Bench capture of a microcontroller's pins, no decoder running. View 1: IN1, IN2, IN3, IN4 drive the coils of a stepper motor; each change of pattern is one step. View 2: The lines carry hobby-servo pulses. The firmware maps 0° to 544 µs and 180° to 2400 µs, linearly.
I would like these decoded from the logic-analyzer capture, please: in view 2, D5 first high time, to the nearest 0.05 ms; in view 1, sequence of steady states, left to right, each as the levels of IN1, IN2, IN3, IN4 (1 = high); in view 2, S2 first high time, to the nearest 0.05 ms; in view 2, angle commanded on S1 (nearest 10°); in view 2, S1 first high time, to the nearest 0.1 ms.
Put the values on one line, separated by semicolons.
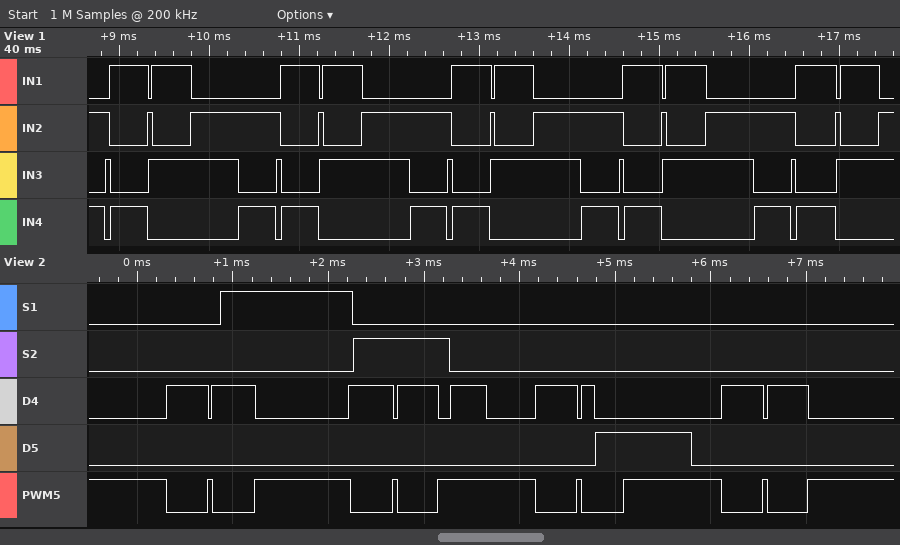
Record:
1.00 ms; 0101 1001 1010 0110 0101 1001 1010 0110 0101 1001 1010 0110 0101 1001 1010 0110 0101 1001 1010 0110; 1.00 ms; 80°; 1.4 ms
